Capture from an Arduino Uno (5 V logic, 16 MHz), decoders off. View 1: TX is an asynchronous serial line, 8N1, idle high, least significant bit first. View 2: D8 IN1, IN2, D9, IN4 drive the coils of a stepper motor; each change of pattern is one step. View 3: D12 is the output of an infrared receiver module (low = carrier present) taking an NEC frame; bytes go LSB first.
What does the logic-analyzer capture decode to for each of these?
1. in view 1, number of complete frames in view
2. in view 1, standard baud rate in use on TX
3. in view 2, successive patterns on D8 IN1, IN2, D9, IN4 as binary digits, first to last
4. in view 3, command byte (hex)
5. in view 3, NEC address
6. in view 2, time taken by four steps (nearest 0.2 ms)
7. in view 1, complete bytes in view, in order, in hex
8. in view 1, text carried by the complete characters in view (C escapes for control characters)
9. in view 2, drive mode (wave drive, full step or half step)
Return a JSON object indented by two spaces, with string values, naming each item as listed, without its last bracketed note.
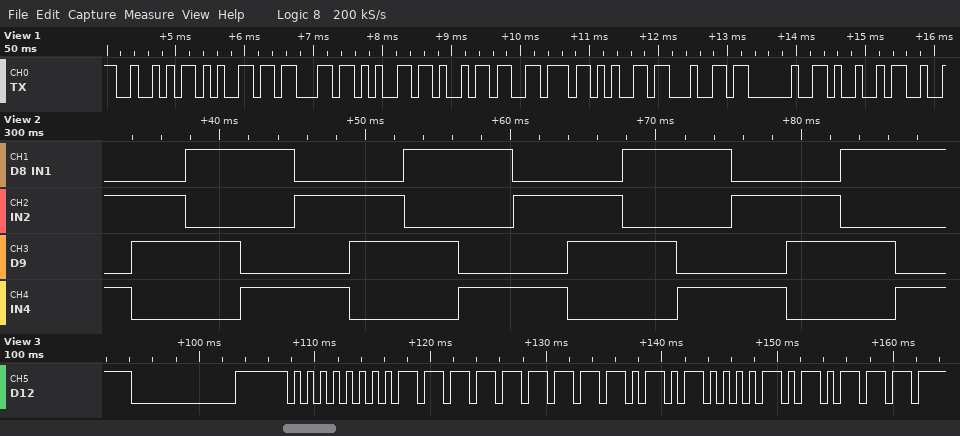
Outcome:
{
  "in view 1, number of complete frames in view": "10",
  "in view 1, standard baud rate in use on TX": "9600 baud",
  "in view 2, successive patterns on D8 IN1, IN2, D9, IN4 as binary digits, first to last": "0101 0110 1010 1001 0101 0110 1010 1001 0101 0110 1010 1001 0101 0110 1010 1001",
  "in view 3, command byte": "0x15",
  "in view 3, NEC address": "0x00",
  "in view 2, time taken by four steps": "15.0 ms",
  "in view 1, complete bytes in view, in order, in hex": "0x52 0x65 0x63 0x65 0x69 0x76 0x65 0x64 0x20 0x49",
  "in view 1, text carried by the complete characters in view": "\"Received I\"",
  "in view 2, drive mode": "full step"
}
